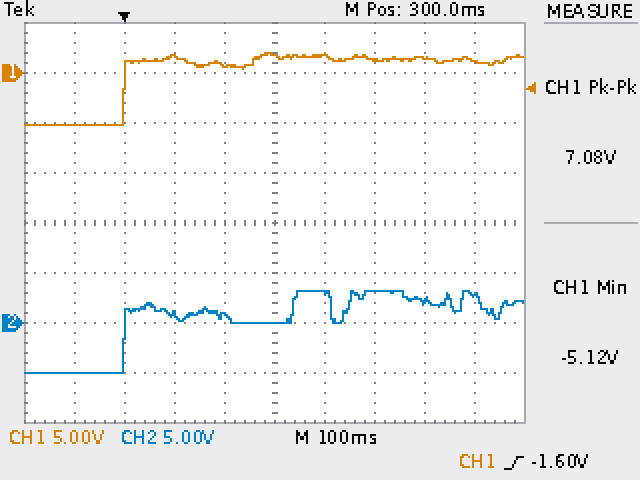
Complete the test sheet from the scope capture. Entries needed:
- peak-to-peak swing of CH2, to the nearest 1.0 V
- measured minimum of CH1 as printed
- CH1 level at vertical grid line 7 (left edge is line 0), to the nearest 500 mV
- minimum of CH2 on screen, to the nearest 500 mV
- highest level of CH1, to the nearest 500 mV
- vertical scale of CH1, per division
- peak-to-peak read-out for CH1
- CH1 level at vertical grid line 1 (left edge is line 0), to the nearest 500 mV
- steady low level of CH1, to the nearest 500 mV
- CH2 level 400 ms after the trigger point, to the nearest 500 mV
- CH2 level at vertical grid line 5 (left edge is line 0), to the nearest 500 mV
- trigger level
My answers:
8.0 V
-5.12 V
1.5 V
-5.0 V
2.0 V
5 V
7.08 V
-5.0 V
-5.0 V
3.0 V
0.0 V
-1.60 V
